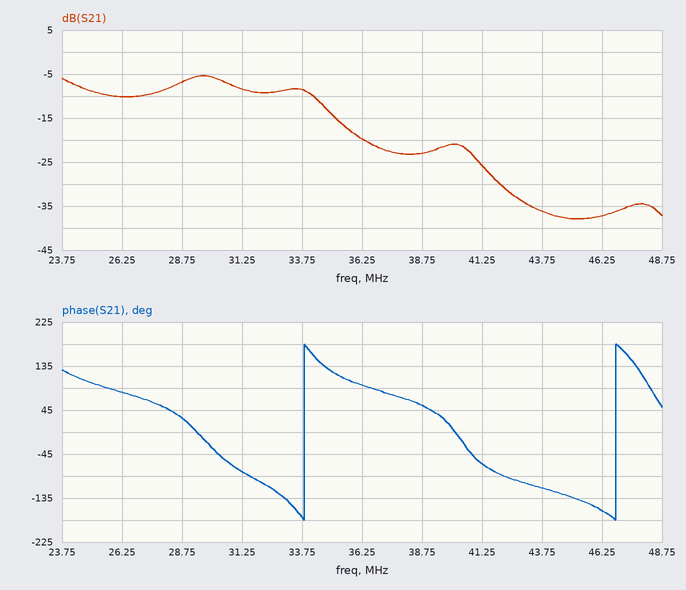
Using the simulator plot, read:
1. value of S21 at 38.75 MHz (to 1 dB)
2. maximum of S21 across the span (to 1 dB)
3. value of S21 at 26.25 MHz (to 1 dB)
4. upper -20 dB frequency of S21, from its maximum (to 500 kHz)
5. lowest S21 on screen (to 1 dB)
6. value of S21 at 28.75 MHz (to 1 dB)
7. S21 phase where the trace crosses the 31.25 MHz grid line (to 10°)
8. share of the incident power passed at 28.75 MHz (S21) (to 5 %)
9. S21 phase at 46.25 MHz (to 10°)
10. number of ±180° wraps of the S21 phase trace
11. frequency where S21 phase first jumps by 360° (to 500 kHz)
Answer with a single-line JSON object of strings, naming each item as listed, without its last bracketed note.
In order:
{"value of S21 at 38.75 MHz": "-23 dB", "maximum of S21 across the span": "-5 dB", "value of S21 at 26.25 MHz": "-10 dB", "upper -20 dB frequency of S21, from its maximum": "41.0 MHz", "lowest S21 on screen": "-38 dB", "value of S21 at 28.75 MHz": "-7 dB", "S21 phase where the trace crosses the 31.25 MHz grid line": "-80°", "share of the incident power passed at 28.75 MHz (S21)": "20 %", "S21 phase at 46.25 MHz": "-160°", "number of ±180° wraps of the S21 phase trace": "2", "frequency where S21 phase first jumps by 360°": "34.0 MHz"}
